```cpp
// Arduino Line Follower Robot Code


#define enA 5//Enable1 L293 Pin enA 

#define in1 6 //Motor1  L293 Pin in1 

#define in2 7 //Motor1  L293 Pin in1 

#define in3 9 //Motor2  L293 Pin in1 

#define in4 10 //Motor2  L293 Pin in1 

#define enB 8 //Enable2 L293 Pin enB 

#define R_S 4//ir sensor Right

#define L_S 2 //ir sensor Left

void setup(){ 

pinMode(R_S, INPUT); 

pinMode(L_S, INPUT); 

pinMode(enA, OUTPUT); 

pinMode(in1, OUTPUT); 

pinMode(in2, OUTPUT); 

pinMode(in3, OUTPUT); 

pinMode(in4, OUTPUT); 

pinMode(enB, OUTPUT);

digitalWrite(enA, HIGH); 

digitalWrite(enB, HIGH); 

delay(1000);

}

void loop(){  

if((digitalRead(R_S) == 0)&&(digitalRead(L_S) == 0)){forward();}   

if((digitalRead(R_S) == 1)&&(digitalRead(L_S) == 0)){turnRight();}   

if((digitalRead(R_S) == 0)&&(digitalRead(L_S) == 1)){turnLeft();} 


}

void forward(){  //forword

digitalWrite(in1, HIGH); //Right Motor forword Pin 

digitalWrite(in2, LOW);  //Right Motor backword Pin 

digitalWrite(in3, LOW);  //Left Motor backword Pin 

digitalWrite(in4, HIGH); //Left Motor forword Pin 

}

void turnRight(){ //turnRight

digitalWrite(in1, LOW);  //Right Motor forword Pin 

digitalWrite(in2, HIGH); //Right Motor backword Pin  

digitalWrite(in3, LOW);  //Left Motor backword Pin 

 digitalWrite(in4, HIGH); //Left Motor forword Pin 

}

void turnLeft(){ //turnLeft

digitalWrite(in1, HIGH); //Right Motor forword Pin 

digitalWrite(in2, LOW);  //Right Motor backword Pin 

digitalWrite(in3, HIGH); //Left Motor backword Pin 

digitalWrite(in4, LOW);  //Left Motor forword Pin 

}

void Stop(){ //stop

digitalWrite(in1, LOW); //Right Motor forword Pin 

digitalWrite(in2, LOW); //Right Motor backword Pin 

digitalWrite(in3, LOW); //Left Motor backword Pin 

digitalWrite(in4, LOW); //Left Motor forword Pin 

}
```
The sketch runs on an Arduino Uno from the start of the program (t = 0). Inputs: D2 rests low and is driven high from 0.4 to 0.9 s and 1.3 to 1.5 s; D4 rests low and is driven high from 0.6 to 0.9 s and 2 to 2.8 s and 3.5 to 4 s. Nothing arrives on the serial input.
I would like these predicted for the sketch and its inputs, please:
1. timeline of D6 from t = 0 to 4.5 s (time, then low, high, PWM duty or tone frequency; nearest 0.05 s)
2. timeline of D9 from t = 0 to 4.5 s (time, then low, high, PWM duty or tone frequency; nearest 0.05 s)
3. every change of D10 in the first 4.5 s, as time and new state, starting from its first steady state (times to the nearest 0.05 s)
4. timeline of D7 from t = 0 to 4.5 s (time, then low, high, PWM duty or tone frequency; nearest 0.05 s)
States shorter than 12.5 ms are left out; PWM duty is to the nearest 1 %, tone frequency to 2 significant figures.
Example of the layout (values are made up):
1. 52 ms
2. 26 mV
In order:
1. 0 s low; 1 s high; 2 s low; 2.8 s high; 3.5 s low; 4 s high
2. 0 s low; 1.3 s high; 1.5 s low
3. 0 s low; 1 s high; 1.3 s low; 1.5 s high
4. 0 s low; 2 s high; 2.8 s low; 3.5 s high; 4 s low
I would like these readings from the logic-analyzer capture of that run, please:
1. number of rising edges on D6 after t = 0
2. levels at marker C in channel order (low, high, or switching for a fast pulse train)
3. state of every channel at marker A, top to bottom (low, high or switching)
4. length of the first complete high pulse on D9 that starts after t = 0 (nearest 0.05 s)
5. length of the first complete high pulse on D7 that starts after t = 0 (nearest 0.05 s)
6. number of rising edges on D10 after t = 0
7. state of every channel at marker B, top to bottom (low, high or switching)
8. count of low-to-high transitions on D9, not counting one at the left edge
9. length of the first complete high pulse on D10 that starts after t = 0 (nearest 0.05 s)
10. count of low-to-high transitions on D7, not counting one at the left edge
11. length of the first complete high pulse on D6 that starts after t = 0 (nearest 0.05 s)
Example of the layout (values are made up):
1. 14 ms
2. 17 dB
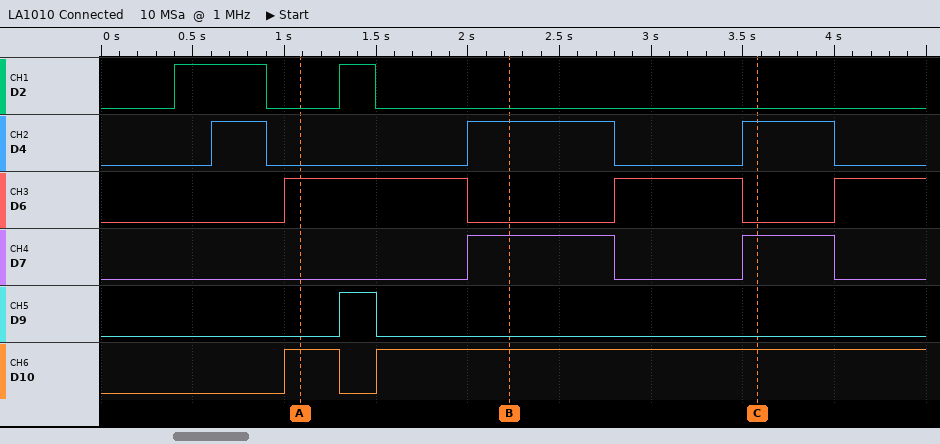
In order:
1. 3
2. D2 low, D4 high, D6 low, D7 high, D9 low, D10 high
3. D2 low, D4 low, D6 high, D7 low, D9 low, D10 high
4. 0.20 s
5. 0.80 s
6. 2
7. D2 low, D4 high, D6 low, D7 high, D9 low, D10 high
8. 1
9. 0.30 s
10. 2
11. 1.00 s
